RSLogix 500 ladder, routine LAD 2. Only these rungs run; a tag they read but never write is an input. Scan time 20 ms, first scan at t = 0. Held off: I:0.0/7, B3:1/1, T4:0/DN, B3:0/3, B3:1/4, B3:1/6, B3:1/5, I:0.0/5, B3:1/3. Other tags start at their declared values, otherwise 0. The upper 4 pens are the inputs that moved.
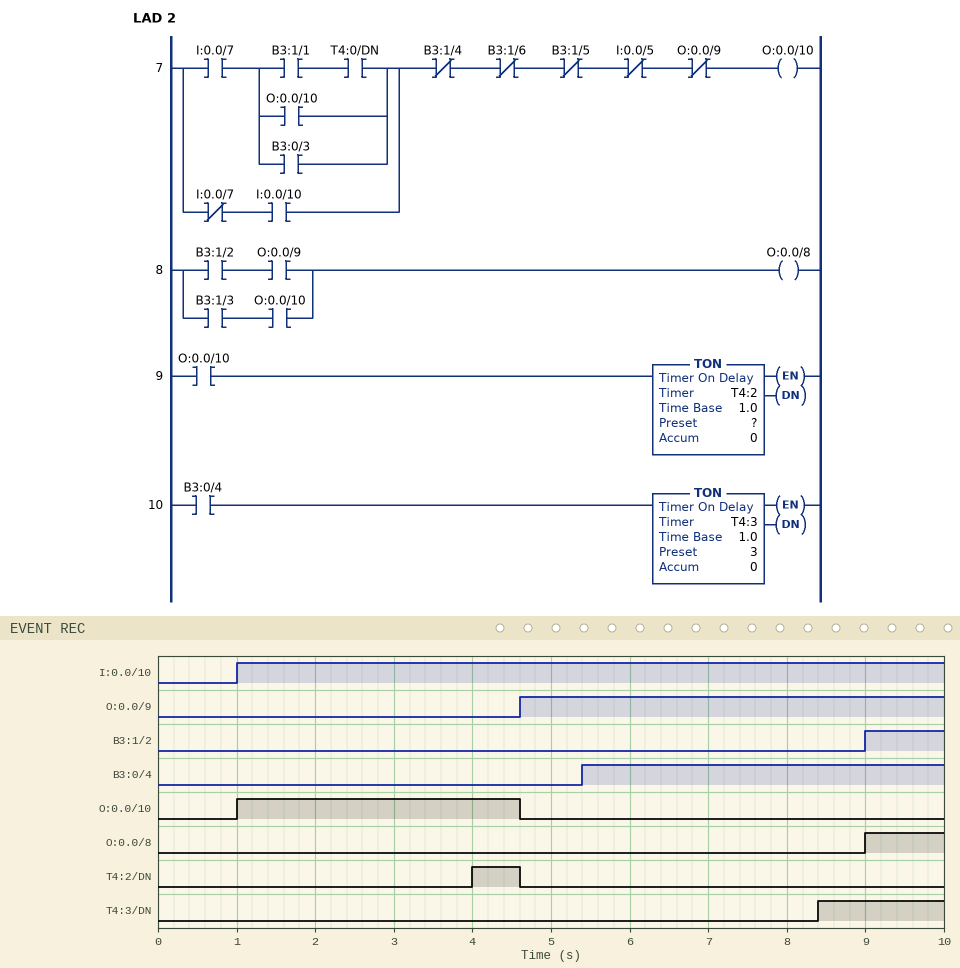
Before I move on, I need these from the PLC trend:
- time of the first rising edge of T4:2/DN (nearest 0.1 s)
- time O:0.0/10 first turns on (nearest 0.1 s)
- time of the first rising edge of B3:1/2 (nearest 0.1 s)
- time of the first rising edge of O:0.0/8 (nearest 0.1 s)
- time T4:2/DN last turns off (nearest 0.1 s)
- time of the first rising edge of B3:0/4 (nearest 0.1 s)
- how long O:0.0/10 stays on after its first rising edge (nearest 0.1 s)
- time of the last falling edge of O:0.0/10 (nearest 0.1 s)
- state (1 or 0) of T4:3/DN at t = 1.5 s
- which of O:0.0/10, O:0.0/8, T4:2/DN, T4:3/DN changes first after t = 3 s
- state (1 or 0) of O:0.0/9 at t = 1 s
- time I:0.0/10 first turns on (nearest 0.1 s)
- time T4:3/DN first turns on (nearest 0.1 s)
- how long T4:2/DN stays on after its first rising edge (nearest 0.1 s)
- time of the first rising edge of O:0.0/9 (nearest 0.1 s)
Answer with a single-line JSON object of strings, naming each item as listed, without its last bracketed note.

{"time of the first rising edge of T4:2/DN": "4.0 s", "time O:0.0/10 first turns on": "1.0 s", "time of the first rising edge of B3:1/2": "9.0 s", "time of the first rising edge of O:0.0/8": "9.0 s", "time T4:2/DN last turns off": "4.6 s", "time of the first rising edge of B3:0/4": "5.4 s", "how long O:0.0/10 stays on after its first rising edge": "3.6 s", "time of the last falling edge of O:0.0/10": "4.6 s", "state (1 or 0) of T4:3/DN at t = 1.5 s": "0", "which of O:0.0/10, O:0.0/8, T4:2/DN, T4:3/DN changes first after t = 3 s": "T4:2/DN", "state (1 or 0) of O:0.0/9 at t = 1 s": "0", "time I:0.0/10 first turns on": "1.0 s", "time T4:3/DN first turns on": "8.4 s", "how long T4:2/DN stays on after its first rising edge": "0.6 s", "time of the first rising edge of O:0.0/9": "4.6 s"}
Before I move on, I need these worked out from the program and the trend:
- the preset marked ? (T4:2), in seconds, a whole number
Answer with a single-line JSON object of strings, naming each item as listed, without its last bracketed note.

{"the preset marked ? (T4:2), in seconds, a whole number": "3 s"}
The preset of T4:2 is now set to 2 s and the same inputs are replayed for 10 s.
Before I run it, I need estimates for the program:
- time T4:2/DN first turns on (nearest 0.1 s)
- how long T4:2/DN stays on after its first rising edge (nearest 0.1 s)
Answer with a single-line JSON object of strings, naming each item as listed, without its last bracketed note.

{"time T4:2/DN first turns on": "3.0 s", "how long T4:2/DN stays on after its first rising edge": "1.6 s"}
